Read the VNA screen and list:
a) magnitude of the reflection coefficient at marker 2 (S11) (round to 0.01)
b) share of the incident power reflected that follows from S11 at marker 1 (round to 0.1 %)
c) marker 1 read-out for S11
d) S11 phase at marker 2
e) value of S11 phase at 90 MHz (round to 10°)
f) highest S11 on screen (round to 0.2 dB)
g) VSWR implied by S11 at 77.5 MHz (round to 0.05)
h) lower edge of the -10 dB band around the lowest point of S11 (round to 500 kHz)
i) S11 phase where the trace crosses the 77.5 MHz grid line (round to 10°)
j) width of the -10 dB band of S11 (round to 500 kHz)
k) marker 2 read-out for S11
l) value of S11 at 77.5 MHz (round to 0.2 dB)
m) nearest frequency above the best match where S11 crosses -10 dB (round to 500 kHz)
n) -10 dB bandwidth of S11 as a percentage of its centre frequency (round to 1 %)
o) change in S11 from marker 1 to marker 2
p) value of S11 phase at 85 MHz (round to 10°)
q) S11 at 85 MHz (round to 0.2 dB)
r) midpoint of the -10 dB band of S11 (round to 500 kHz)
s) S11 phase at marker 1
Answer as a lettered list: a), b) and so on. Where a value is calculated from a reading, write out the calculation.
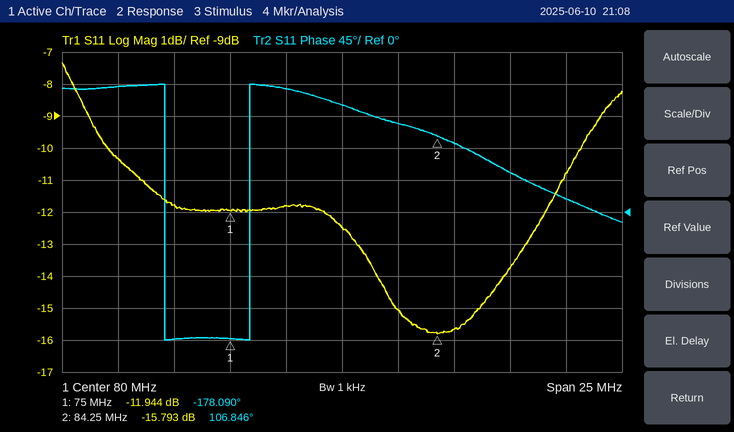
a) 10^(-15.793/20) ≈ 0.16
b) 10^(-11.944/10) ≈ 6.4 %
c) -11.944 dB
d) 106.846°
e) 20°
f) -7.4 dB
g) |Γ| = 10^(-11.8/20) = 0.2570; VSWR = (1 + 0.2570)/(1 − 0.2570) ≈ 1.69, so 1.70 to the nearest 0.05
h) 69.5 MHz
i) 170°
j) 90.5 MHz − 69.5 MHz = 21.0 MHz
k) -15.793 dB
l) -11.8 dB
m) 90.5 MHz
n) 21 MHz / 80 MHz ≈ 26 %
o) -15.793 − (-11.944) = -3.849 dB
p) 100°
q) -15.6 dB
r) 80.0 MHz
s) -178.090°
